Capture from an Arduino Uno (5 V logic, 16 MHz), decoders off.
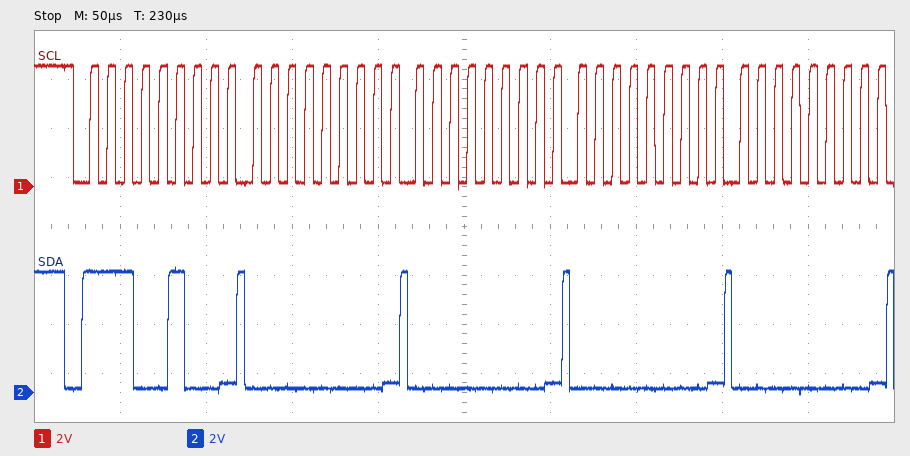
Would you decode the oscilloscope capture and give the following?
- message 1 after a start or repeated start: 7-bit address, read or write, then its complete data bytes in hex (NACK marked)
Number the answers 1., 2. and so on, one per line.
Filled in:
1. 0x72 write: 00 00 00 00
